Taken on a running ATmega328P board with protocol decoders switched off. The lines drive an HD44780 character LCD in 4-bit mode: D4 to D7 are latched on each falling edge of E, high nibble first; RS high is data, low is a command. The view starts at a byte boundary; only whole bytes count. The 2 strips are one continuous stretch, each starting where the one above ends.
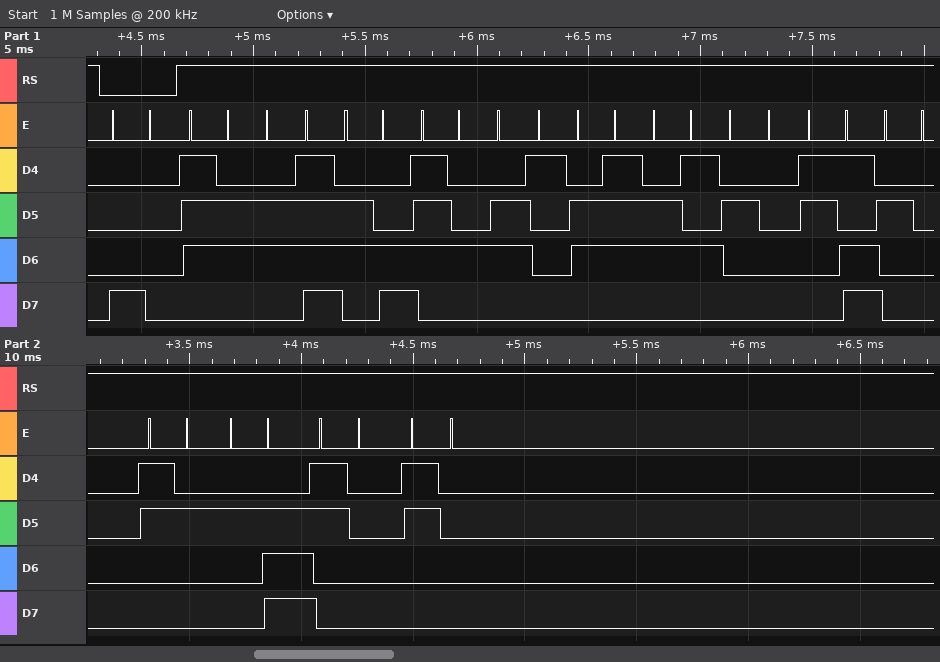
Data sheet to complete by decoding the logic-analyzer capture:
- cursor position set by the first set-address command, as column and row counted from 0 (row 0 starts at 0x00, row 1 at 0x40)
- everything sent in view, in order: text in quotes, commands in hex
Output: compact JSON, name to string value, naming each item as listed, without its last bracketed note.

{"cursor position set by the first set-address command, as column and row counted from 0": "column 0, row 0", "everything sent in view, in order: text in quotes, commands in hex": "0x80 \"voltage = 2.00\""}
